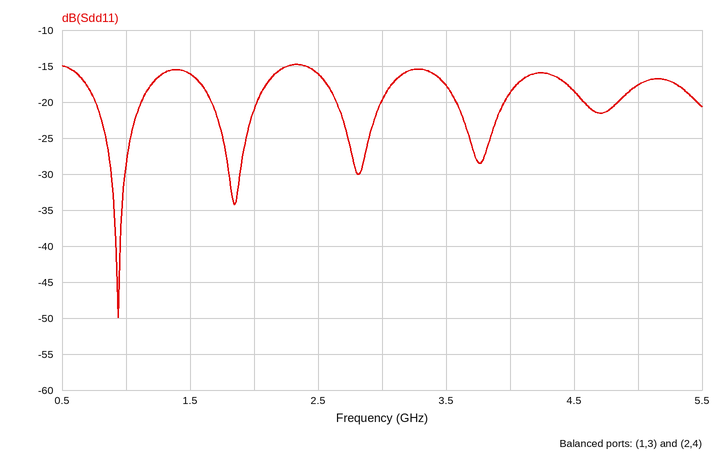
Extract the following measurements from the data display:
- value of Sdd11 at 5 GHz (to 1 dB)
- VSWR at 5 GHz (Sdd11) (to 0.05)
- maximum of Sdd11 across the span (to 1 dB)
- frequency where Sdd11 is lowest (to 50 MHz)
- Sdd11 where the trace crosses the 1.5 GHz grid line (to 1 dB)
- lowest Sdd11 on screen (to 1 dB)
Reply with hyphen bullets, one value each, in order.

- -18 dB
- 1.30
- -15 dB
- 950 MHz
- -16 dB
- -50 dB
